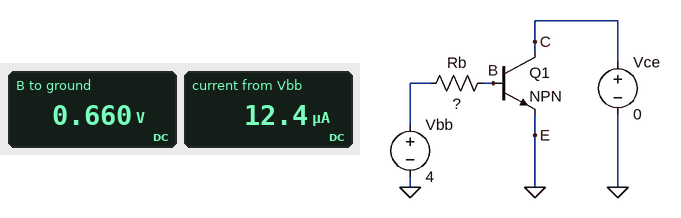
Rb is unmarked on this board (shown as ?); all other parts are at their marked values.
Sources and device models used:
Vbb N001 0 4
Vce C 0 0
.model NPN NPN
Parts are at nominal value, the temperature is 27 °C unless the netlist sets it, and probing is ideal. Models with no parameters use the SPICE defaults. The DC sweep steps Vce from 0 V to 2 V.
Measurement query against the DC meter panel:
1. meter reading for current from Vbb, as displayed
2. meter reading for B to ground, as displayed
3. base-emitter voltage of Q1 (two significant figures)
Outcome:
12.4 µA
0.660 V
660 mV
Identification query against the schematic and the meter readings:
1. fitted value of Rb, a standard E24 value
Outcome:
270 kΩ
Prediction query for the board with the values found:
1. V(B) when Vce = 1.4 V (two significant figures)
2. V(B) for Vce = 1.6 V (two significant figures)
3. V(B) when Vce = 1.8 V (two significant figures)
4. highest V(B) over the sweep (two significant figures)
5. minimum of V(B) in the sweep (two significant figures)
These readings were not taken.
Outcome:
780 mV
780 mV
780 mV
780 mV
660 mV
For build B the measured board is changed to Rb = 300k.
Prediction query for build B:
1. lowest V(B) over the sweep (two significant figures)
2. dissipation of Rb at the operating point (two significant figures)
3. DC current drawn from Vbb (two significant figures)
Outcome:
660 mV
37 µW
11 µA
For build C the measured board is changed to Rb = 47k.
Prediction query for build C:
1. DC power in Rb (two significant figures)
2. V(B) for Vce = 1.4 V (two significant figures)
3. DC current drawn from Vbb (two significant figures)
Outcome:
230 µW
820 mV
70 µA
